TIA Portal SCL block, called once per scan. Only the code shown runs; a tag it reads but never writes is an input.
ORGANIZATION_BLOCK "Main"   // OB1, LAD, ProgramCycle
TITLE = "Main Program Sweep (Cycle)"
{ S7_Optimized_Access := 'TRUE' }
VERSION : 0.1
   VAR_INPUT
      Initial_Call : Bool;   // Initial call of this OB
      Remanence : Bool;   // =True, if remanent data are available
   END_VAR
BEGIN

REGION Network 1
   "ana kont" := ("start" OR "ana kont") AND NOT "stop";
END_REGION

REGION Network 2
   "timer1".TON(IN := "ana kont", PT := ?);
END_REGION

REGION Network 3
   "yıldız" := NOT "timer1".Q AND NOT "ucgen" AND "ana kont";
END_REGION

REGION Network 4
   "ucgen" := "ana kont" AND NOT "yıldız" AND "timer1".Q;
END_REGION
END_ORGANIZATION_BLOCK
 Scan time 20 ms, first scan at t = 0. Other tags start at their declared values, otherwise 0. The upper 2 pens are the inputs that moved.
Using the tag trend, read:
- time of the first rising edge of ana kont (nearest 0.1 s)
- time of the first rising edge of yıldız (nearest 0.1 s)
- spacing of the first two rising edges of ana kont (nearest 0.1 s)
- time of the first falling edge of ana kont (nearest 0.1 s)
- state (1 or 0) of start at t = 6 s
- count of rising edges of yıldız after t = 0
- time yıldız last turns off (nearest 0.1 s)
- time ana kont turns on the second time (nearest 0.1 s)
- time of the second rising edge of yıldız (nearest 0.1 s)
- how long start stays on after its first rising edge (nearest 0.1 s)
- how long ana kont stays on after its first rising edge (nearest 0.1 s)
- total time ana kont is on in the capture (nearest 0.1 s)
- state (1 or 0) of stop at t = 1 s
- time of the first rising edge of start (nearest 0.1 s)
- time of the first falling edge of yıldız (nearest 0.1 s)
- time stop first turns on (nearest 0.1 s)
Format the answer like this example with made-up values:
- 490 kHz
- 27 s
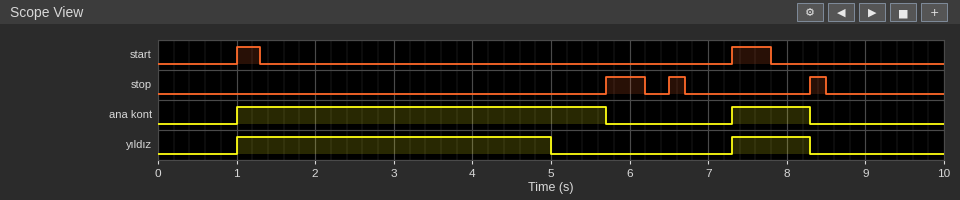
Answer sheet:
- 1.0 s
- 1.0 s
- 6.3 s
- 5.7 s
- 0
- 2
- 8.3 s
- 7.3 s
- 7.3 s
- 0.3 s
- 4.7 s
- 5.7 s
- 0
- 1.0 s
- 5.0 s
- 5.7 s
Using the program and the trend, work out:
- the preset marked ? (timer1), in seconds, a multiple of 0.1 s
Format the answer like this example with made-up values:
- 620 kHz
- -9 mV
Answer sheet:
- 4.0 s
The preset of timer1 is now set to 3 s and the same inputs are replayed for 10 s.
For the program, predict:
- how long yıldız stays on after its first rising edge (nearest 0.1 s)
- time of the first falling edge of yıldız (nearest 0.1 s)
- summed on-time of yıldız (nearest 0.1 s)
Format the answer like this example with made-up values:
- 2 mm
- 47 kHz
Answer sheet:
- 3.0 s
- 4.0 s
- 4.0 s
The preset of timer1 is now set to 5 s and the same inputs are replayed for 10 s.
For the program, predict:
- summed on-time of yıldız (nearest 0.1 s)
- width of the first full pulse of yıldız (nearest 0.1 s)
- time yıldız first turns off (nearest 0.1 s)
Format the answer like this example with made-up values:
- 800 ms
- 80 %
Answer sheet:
- 5.7 s
- 4.7 s
- 5.7 s
